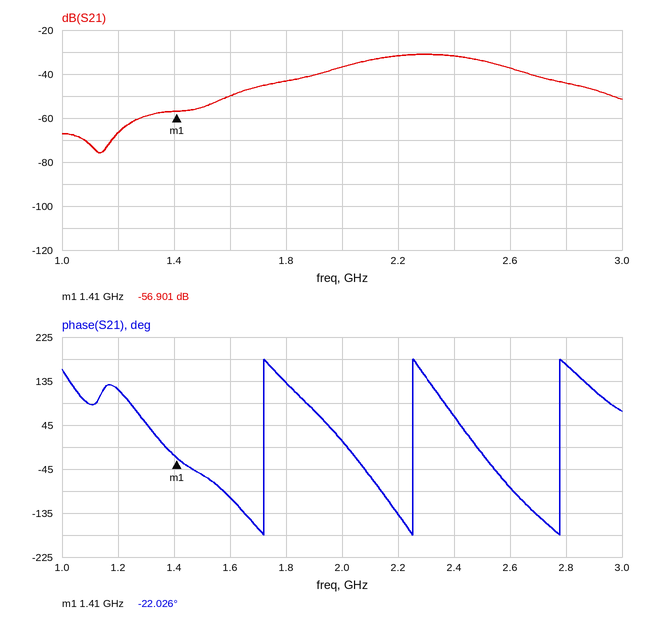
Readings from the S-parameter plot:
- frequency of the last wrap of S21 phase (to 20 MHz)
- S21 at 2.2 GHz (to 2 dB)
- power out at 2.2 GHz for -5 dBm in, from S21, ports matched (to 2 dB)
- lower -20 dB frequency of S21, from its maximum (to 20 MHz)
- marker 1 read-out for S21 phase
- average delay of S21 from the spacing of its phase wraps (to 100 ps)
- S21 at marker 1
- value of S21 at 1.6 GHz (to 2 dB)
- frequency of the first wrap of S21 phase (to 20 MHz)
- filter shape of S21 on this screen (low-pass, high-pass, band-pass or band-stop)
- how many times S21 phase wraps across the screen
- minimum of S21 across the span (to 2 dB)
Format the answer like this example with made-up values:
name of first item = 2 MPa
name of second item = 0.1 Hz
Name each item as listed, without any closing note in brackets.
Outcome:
frequency of the last wrap of S21 phase = 2.78 GHz
S21 at 2.2 GHz = -32 dB
power out at 2.2 GHz for -5 dBm in, from S21, ports matched = -36 dBm
lower -20 dB frequency of S21, from its maximum = 1.58 GHz
marker 1 read-out for S21 phase = -22.026°
average delay of S21 from the spacing of its phase wraps = 1.9 ns
S21 at marker 1 = -56.901 dB
value of S21 at 1.6 GHz = -50 dB
frequency of the first wrap of S21 phase = 1.72 GHz
filter shape of S21 on this screen = band-pass
how many times S21 phase wraps across the screen = 3
minimum of S21 across the span = -76 dB
